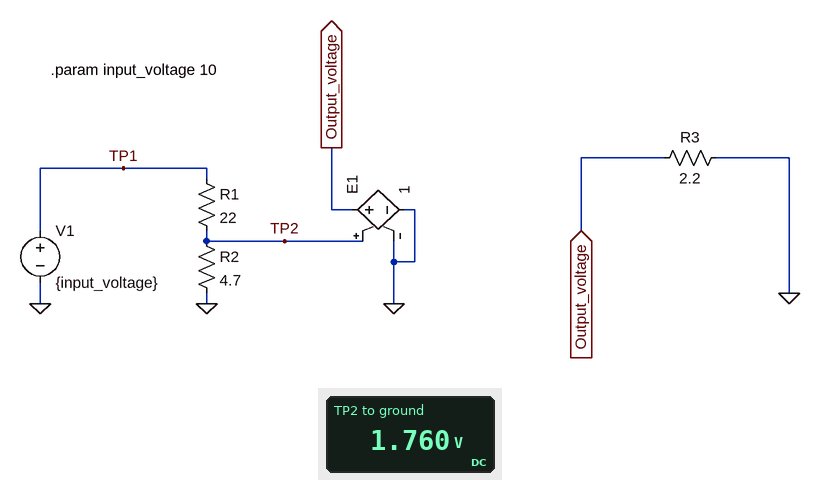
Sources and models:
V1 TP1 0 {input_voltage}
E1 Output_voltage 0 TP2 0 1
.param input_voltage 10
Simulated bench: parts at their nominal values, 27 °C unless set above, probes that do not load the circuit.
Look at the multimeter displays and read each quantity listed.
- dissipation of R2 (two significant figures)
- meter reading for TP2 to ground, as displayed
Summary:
660 mW
1.760 V
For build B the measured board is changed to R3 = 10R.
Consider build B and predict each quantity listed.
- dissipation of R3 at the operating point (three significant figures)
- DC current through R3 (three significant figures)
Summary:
310 mW
176 mA
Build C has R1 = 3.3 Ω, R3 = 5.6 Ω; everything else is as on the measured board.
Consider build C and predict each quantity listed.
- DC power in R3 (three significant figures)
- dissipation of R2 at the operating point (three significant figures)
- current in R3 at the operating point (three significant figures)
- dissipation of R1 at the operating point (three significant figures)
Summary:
6.16 W
7.34 W
1.05 A
5.16 W
